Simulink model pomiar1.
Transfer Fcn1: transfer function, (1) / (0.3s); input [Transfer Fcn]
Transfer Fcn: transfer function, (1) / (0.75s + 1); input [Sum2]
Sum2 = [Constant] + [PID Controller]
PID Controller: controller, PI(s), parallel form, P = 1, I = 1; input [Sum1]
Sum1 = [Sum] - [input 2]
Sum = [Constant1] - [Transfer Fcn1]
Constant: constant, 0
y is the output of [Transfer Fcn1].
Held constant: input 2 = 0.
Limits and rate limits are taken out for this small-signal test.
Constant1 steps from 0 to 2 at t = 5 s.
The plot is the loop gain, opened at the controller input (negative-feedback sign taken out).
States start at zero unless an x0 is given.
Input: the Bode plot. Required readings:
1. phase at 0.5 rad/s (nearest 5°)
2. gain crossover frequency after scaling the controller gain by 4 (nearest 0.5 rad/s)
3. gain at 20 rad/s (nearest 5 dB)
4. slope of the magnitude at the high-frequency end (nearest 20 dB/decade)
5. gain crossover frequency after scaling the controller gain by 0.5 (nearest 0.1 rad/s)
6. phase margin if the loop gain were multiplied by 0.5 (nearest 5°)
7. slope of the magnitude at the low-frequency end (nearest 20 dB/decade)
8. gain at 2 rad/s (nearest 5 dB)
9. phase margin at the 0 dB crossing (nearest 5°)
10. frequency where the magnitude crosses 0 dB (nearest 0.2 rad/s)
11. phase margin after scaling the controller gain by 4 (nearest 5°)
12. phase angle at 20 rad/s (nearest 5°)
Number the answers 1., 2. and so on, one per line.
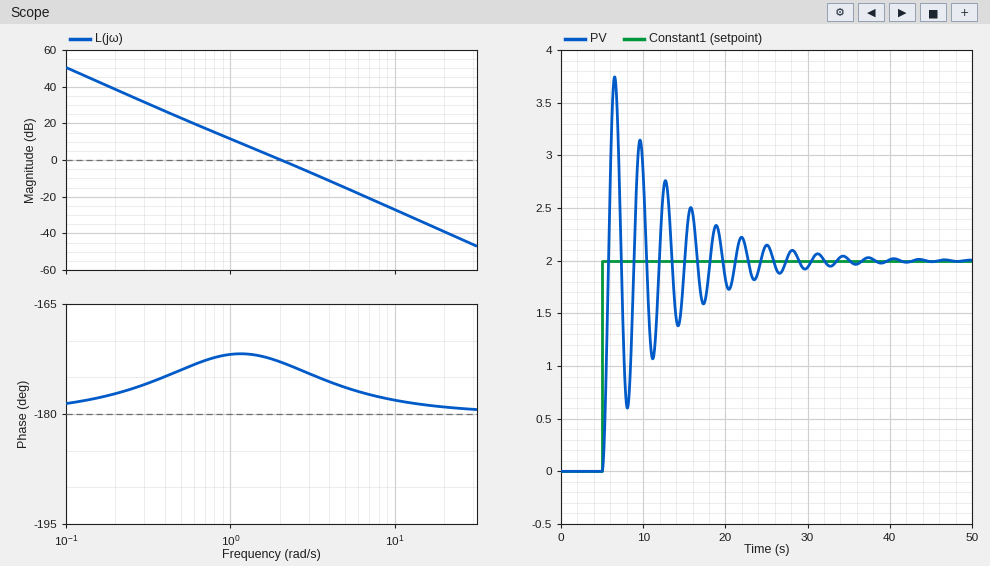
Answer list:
1. -175°
2. 4.0 rad/s
3. -40 dB
4. -40 dB/decade
5. 1.4 rad/s
6. 10°
7. -40 dB/decade
8. 0 dB
9. 5°
10. 2.0 rad/s
11. 5°
12. -180°
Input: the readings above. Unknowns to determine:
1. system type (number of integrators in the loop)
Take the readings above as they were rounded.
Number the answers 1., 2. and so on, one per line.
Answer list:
1. 2
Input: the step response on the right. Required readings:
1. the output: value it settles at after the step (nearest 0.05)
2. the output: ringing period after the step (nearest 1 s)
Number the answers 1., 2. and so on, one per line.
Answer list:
1. 2.00
2. 3 s
